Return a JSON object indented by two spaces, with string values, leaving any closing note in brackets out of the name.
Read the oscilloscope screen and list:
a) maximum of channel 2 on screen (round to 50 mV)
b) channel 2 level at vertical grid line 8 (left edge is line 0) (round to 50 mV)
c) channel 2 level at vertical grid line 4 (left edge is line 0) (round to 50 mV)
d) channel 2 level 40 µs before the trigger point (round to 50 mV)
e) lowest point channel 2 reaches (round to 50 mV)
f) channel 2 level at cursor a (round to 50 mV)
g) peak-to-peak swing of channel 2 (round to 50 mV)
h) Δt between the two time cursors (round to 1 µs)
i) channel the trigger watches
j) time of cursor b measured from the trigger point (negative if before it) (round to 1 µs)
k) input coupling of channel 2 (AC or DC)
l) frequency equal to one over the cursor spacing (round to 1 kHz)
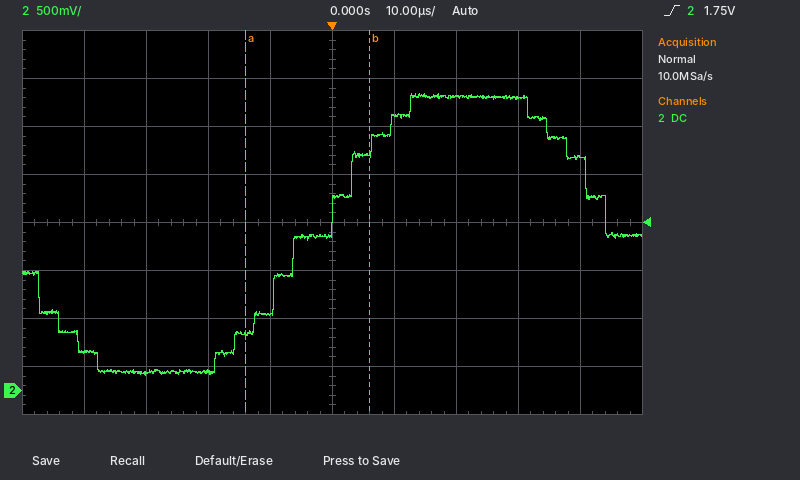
{
  "maximum of channel 2 on screen": "3.10 V",
  "channel 2 level at vertical grid line 8 (left edge is line 0)": "3.05 V",
  "channel 2 level at vertical grid line 4 (left edge is line 0)": "800 mV",
  "channel 2 level 40 µs before the trigger point": "400 mV",
  "lowest point channel 2 reaches": "150 mV",
  "channel 2 level at cursor a": "600 mV",
  "peak-to-peak swing of channel 2": "2.95 V",
  "Δt between the two time cursors": "20 µs",
  "channel the trigger watches": "channel 2",
  "time of cursor b measured from the trigger point (negative if before it)": "+6 µs",
  "input coupling of channel 2": "DC",
  "frequency equal to one over the cursor spacing": "50 kHz"
}
